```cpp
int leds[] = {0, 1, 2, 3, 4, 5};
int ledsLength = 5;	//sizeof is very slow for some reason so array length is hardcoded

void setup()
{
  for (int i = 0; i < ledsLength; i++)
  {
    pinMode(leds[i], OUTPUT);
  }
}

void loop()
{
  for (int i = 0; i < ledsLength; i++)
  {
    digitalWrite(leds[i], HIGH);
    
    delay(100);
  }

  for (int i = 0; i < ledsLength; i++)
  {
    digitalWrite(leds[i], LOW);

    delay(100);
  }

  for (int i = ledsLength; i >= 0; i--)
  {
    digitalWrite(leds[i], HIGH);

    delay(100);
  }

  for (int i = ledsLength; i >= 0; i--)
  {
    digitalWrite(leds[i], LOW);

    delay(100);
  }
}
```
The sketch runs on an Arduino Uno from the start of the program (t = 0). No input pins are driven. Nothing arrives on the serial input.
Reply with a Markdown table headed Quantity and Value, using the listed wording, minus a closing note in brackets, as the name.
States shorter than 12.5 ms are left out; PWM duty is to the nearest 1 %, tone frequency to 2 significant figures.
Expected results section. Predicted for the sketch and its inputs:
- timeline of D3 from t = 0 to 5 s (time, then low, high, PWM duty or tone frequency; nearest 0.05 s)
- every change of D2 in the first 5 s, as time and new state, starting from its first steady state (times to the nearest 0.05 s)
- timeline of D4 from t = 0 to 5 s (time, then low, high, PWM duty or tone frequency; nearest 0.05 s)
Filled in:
| Quantity | Value |
|---|---|
| timeline of D3 from t = 0 to 5 s | 0 s low; 0.3 s high; 0.8 s low; 1.2 s high; 1.8 s low; 2.5 s high; 3 s low; 3.4 s high; 4 s low; 4.7 s high |
| every change of D2 in the first 5 s, as time and new state, starting from its first steady state | 0 s low; 0.2 s high; 0.7 s low; 1.3 s high; 1.9 s low; 2.4 s high; 2.9 s low; 3.5 s high; 4.1 s low; 4.6 s high |
| timeline of D4 from t = 0 to 5 s | 0 s low; 0.4 s high; 0.9 s low; 1.1 s high; 1.7 s low; 2.6 s high; 3.1 s low; 3.3 s high; 3.9 s low; 4.8 s high |
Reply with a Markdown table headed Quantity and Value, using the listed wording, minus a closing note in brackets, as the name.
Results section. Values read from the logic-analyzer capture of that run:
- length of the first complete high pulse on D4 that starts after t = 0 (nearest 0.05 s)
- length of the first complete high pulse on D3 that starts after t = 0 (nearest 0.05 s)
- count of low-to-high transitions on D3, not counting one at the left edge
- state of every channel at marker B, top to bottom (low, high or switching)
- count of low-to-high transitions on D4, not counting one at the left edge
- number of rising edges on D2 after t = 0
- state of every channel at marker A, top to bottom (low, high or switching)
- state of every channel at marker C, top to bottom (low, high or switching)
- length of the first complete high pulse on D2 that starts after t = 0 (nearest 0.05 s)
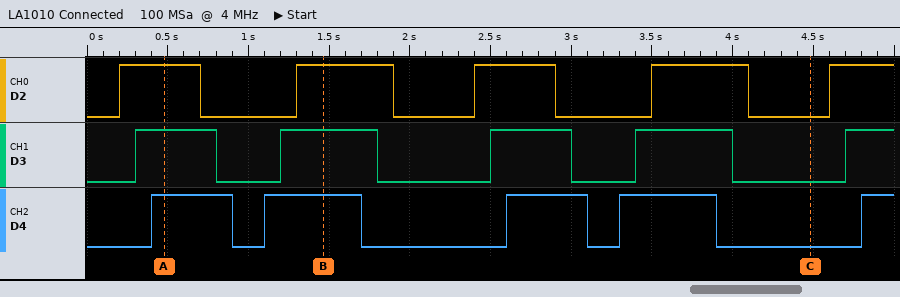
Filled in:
| Quantity | Value |
|---|---|
| length of the first complete high pulse on D4 that starts after t = 0 | 0.50 s |
| length of the first complete high pulse on D3 that starts after t = 0 | 0.50 s |
| count of low-to-high transitions on D3, not counting one at the left edge | 5 |
| state of every channel at marker B, top to bottom | D2 high, D3 high, D4 high |
| count of low-to-high transitions on D4, not counting one at the left edge | 5 |
| number of rising edges on D2 after t = 0 | 5 |
| state of every channel at marker A, top to bottom | D2 high, D3 high, D4 high |
| state of every channel at marker C, top to bottom | D2 low, D3 low, D4 low |
| length of the first complete high pulse on D2 that starts after t = 0 | 0.50 s |
